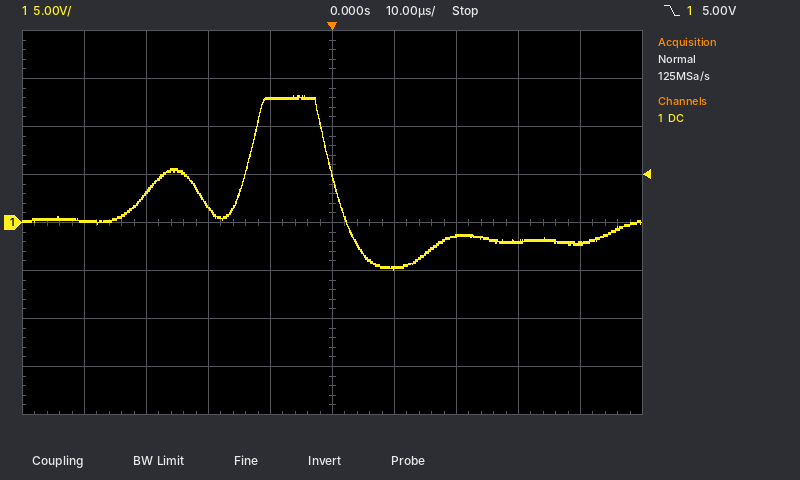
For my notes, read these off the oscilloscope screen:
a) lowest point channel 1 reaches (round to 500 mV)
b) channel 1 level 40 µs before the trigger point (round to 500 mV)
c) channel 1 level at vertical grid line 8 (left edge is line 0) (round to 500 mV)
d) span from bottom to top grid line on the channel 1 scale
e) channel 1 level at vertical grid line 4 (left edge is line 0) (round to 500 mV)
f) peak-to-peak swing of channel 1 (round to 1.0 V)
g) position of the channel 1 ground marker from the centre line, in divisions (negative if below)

-5.0 V
0.0 V
-2.0 V
40 V
13.0 V
18.0 V
0.0 div
